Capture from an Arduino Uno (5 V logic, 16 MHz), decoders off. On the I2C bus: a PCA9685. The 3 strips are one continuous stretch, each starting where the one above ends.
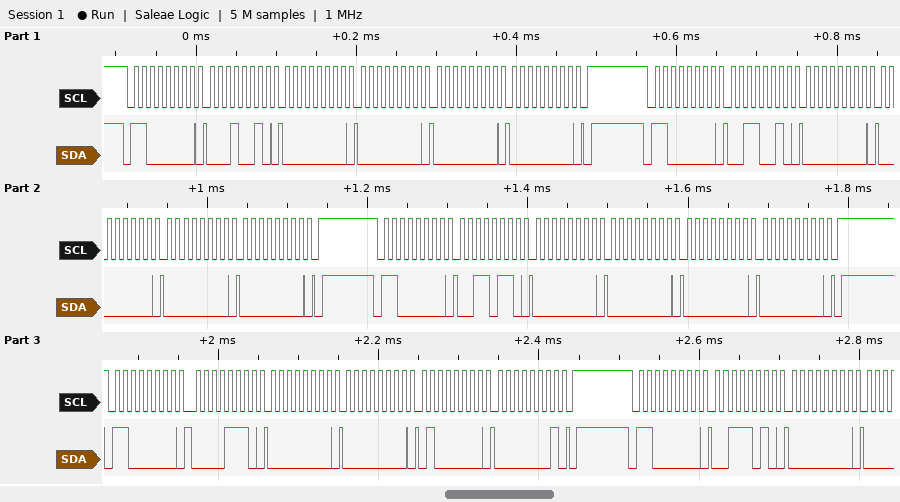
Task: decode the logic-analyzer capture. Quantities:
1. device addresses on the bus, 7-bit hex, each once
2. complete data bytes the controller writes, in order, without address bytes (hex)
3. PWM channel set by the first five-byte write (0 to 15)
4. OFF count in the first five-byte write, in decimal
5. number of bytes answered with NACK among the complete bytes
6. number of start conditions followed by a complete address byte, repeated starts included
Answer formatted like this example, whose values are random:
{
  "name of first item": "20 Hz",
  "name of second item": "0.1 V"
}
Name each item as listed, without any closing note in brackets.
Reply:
{
  "device addresses on the bus, 7-bit hex, each once": "0x60",
  "complete data bytes the controller writes, in order, without address bytes": "12 00 00 00 00 32 00 00 00 00 36 00 00 00 00 0E 00 00 40 01 3A 00",
  "PWM channel set by the first five-byte write": "3",
  "OFF count in the first five-byte write, in decimal": "0",
  "number of bytes answered with NACK among the complete bytes": "0",
  "number of start conditions followed by a complete address byte, repeated starts included": "5"
}
